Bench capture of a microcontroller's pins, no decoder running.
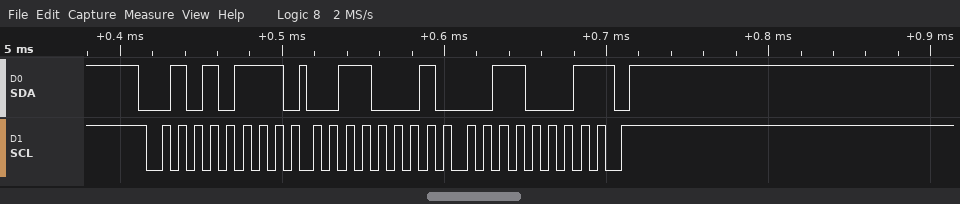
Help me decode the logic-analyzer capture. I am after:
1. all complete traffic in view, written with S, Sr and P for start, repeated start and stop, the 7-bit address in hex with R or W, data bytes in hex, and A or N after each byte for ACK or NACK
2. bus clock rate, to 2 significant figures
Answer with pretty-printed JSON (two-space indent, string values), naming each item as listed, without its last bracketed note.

{
  "all complete traffic in view, written with S, Sr and P for start, repeated start and stop, the 7-bit address in hex with R or W, data bytes in hex, and A or N after each byte for ACK or NACK": "S 2BR A 31 A 31 N P",
  "bus clock rate, to 2 significant figures": "100 kHz"
}
